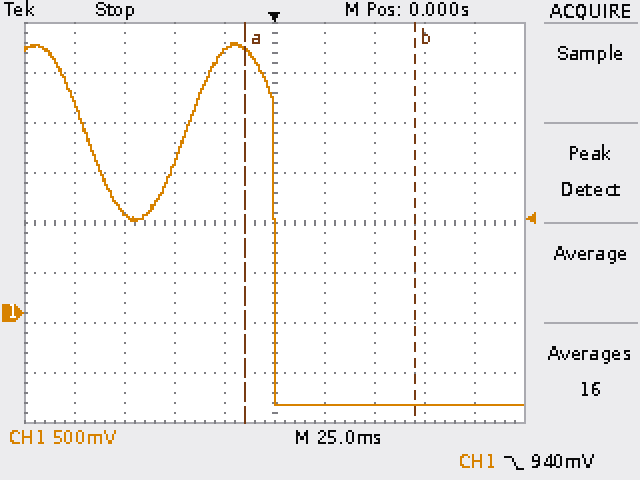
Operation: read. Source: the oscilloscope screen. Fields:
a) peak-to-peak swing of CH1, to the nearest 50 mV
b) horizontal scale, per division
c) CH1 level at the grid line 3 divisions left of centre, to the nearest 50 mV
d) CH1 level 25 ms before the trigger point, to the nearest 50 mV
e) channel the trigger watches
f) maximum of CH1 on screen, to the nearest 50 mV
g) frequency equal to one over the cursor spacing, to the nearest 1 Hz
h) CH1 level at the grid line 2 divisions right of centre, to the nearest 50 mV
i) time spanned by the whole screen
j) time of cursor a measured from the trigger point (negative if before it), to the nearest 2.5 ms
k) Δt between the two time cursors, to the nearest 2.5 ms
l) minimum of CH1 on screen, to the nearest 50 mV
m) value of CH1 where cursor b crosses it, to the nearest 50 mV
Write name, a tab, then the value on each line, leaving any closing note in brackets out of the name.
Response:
peak-to-peak swing of CH1, to the nearest 50 mV	3.60 V
horizontal scale, per division	25 ms
CH1 level at the grid line 3 divisions left of centre, to the nearest 50 mV	1.00 V
CH1 level 25 ms before the trigger point, to the nearest 50 mV	2.60 V
channel the trigger watches	CH1
maximum of CH1 on screen, to the nearest 50 mV	2.70 V
frequency equal to one over the cursor spacing, to the nearest 1 Hz	12 Hz
CH1 level at the grid line 2 divisions right of centre, to the nearest 50 mV	-900 mV
time spanned by the whole screen	250 ms
time of cursor a measured from the trigger point (negative if before it), to the nearest 2.5 ms	-15.0 ms
Δt between the two time cursors, to the nearest 2.5 ms	85.0 ms
minimum of CH1 on screen, to the nearest 50 mV	-900 mV
value of CH1 where cursor b crosses it, to the nearest 50 mV	-900 mV
